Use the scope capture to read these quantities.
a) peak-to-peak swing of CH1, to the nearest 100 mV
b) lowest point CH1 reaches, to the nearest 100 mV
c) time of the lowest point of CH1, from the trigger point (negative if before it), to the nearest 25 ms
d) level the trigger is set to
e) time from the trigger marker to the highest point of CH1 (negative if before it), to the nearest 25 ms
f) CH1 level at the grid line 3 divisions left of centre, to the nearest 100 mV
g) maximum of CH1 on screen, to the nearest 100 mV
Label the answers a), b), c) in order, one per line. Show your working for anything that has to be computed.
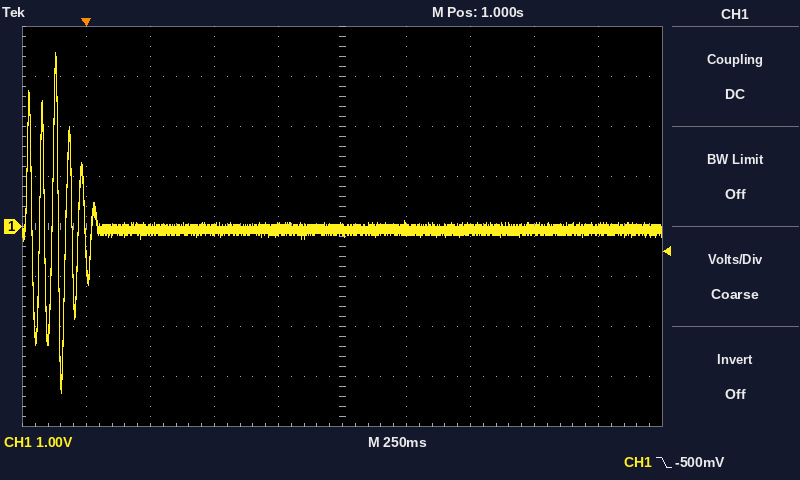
a) 3.5 V − (-3.3 V) = 6.8 V
b) -3.3 V
c) -100 ms
d) -500 mV
e) -125 ms
f) -100 mV
g) 3.5 V
